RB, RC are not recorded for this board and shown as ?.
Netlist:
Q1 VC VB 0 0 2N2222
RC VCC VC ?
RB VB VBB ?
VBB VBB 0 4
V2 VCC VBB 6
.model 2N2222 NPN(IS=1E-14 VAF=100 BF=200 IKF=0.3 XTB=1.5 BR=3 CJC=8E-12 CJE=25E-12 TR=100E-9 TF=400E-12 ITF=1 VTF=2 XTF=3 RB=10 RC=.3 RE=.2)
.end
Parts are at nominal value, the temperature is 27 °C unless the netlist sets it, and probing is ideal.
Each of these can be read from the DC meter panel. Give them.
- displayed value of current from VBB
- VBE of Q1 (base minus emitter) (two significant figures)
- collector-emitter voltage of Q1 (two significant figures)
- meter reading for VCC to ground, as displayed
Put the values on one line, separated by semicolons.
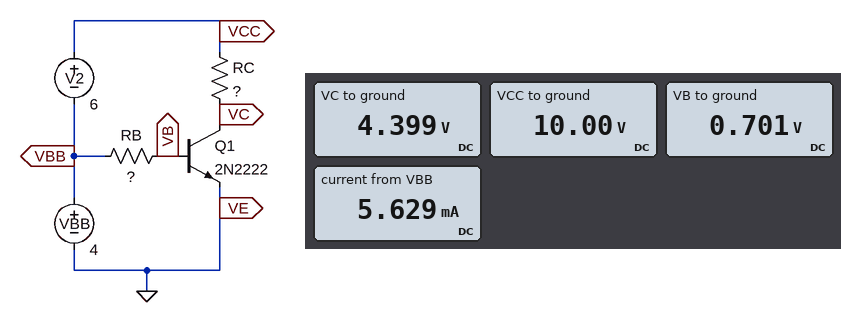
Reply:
5.629 mA; 700 mV; 4.4 V; 10.00 V
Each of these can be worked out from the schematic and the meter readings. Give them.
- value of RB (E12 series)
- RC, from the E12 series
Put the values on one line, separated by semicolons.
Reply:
120 kΩ; 1 kΩ
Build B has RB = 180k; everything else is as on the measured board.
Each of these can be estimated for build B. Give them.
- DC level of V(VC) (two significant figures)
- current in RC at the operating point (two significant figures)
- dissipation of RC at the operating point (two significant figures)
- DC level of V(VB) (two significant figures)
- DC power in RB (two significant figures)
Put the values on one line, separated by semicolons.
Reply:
6.2 V; 3.8 mA; 15 mW; 690 mV; 61 µW
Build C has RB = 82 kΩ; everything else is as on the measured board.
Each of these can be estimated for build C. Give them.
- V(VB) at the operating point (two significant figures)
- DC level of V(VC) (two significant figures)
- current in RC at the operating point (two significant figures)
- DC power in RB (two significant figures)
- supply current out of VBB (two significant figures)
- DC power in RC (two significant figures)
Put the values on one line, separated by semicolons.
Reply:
710 mV; 2.1 V; 7.9 mA; 130 µW; 8.0 mA; 63 mW
